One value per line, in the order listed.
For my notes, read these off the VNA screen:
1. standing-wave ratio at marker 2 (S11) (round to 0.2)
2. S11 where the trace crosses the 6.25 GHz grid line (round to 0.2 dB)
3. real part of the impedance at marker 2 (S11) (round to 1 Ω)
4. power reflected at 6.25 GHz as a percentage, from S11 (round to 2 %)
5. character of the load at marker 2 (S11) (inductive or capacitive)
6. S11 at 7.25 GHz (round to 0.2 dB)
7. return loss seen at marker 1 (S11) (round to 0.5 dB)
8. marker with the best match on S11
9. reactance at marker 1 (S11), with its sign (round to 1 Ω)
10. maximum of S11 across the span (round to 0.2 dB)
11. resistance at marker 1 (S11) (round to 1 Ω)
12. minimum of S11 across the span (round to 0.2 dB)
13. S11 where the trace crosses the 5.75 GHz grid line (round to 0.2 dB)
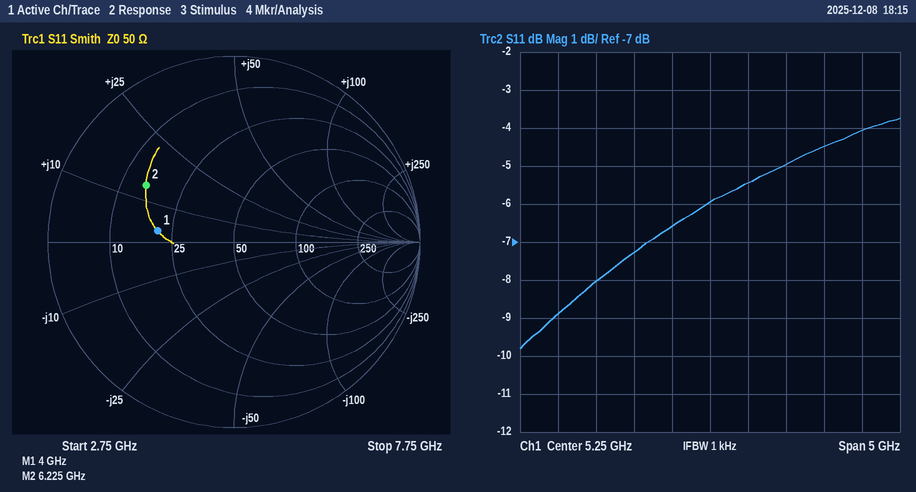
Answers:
3.6
-5.0 dB
15 Ω
32 %
inductive
-4.0 dB
7.5 dB
marker 1
+3 Ω
-3.8 dB
21 Ω
-9.8 dB
-5.4 dB
